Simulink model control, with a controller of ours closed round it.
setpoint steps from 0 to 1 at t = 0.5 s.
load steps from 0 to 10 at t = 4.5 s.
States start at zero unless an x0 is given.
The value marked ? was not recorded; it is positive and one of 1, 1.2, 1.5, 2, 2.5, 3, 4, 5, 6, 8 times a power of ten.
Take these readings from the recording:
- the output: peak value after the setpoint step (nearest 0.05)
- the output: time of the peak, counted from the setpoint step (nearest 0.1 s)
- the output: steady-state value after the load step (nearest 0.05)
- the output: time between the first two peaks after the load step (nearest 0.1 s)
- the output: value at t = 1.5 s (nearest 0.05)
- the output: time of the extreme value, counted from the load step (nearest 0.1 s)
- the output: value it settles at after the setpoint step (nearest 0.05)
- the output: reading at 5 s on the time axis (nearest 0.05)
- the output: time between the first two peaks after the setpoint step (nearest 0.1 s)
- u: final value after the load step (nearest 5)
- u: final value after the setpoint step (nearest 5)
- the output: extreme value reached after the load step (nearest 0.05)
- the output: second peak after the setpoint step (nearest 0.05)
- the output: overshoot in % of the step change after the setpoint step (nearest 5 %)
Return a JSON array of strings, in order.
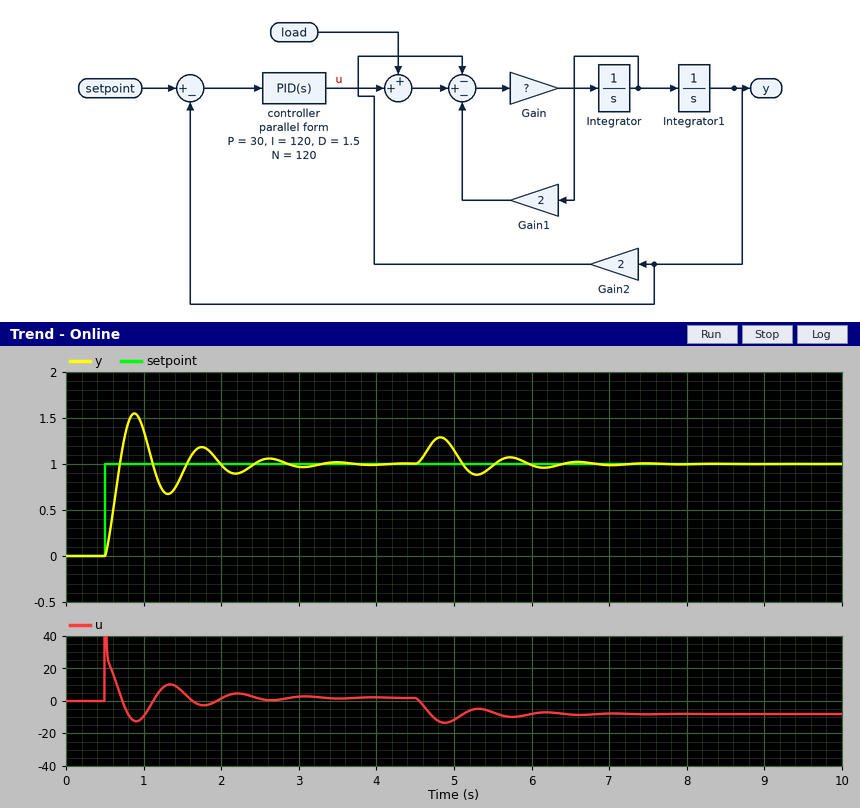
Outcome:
["1.55", "0.4 s", "1.00", "0.9 s", "0.90", "0.3 s", "1.00", "1.15", "0.9 s", "-10", "0", "1.30", "1.20", "55 %"]
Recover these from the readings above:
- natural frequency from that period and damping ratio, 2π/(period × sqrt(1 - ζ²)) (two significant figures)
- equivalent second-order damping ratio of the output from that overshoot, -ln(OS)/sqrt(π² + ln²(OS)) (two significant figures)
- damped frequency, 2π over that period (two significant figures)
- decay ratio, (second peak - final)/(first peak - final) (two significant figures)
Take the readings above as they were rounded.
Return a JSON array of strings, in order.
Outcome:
["7.1 rad/s", "0.19", "7.0 rad/s", "0.36"]
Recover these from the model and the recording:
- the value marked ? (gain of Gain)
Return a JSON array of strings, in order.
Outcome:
["2"]
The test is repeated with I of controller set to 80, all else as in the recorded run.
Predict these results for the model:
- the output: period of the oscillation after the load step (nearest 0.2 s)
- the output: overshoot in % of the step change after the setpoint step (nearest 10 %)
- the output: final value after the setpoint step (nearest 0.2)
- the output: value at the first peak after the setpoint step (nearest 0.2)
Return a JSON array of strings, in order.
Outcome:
["1.0 s", "40 %", "1.0", "1.4"]
